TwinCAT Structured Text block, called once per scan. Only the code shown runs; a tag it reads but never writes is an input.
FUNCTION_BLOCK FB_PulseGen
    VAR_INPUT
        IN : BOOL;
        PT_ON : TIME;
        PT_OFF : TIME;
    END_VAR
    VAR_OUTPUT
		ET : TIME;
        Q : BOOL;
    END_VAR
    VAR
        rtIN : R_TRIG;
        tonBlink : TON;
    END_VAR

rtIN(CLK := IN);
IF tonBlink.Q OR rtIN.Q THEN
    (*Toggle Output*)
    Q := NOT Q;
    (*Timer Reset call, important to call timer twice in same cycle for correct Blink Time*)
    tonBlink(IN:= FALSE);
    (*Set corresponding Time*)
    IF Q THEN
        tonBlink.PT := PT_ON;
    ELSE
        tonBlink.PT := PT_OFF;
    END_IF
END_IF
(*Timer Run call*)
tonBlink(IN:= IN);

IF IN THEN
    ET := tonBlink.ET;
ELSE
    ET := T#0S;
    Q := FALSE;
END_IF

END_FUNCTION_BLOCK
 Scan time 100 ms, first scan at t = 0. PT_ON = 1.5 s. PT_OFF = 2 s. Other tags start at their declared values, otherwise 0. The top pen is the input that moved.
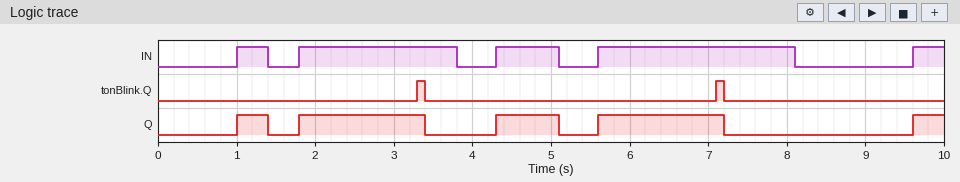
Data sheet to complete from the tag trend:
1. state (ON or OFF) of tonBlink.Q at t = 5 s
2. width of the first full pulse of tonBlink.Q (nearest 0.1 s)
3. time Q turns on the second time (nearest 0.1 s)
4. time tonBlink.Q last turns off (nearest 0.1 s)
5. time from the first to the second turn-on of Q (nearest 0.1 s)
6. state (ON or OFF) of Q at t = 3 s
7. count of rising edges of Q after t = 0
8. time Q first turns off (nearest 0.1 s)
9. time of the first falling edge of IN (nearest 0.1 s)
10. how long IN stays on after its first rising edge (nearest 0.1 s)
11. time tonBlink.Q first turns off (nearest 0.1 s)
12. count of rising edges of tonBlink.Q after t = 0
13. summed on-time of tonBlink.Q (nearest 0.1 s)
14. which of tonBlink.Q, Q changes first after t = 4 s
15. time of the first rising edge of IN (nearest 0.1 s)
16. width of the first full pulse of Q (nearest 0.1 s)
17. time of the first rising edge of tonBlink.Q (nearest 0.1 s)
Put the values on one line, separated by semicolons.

OFF; 0.1 s; 1.8 s; 7.2 s; 0.8 s; ON; 5; 1.4 s; 1.4 s; 0.4 s; 3.4 s; 2; 0.2 s; Q; 1.0 s; 0.4 s; 3.3 s
